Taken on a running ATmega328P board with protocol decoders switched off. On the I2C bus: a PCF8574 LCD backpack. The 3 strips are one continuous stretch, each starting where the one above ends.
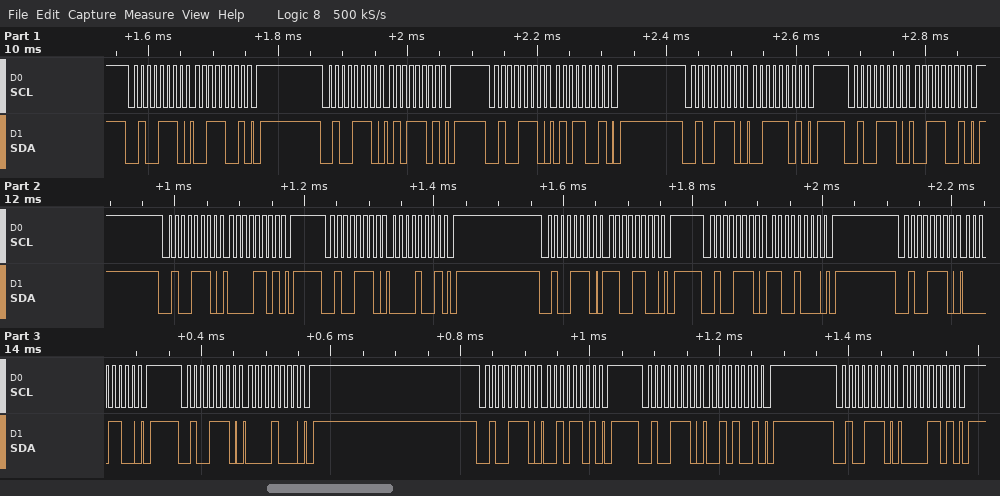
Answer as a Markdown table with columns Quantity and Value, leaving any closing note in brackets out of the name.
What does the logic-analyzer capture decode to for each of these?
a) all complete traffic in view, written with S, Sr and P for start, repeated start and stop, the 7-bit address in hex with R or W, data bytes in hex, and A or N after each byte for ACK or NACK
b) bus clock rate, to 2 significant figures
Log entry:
| Quantity | Value |
|---|---|
| all complete traffic in view, written with S, Sr and P for start, repeated start and stop, the 7-bit address in hex with R or W, data bytes in hex, and A or N after each byte for ACK or NACK | S 27W A 39 A P S 27W A 5D A P S 27W A 59 A P S 27W A 3D A P S 27W A 39 A P S 27W A 0D A P S 27W A 09 A P S 27W A CC A P S 27W A C8 A P S 27W A 0C A P S 27W A 08 A P S 27W A 2D A P S 27W A 29 A P S 27W A 0D A P |
| bus clock rate, to 2 significant figures | 100 kHz |
